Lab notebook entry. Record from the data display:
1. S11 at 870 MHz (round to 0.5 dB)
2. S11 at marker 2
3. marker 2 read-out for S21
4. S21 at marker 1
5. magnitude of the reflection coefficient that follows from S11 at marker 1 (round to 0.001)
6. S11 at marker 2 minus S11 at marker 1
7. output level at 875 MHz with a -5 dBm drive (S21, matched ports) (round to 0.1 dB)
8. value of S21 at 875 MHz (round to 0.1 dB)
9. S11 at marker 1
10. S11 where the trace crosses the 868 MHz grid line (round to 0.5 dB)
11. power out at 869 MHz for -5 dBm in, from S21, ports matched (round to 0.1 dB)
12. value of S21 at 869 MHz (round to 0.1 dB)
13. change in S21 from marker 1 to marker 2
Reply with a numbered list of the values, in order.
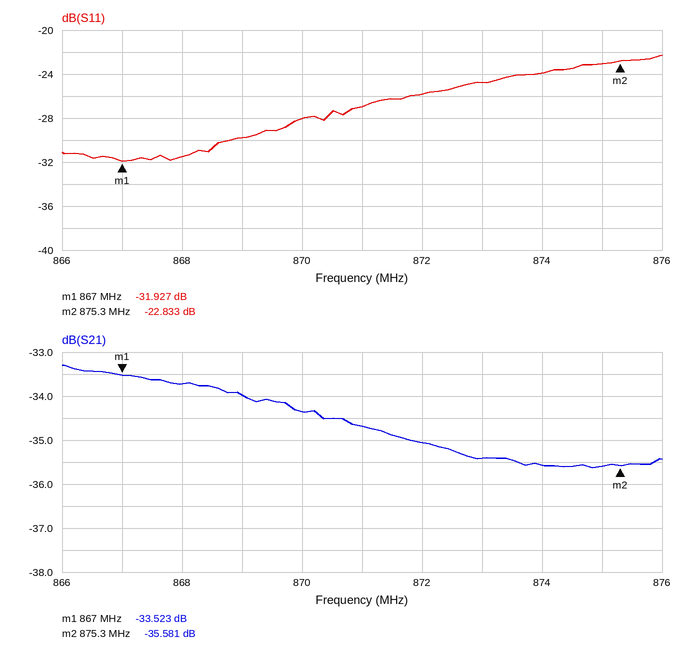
1. -28.0 dB
2. -22.833 dB
3. -35.581 dB
4. -33.523 dB
5. 0.025
6. 9.094 dB
7. -40.6 dBm
8. -35.6 dB
9. -31.927 dB
10. -31.5 dB
11. -39.0 dBm
12. -34.0 dB
13. -2.058 dB
